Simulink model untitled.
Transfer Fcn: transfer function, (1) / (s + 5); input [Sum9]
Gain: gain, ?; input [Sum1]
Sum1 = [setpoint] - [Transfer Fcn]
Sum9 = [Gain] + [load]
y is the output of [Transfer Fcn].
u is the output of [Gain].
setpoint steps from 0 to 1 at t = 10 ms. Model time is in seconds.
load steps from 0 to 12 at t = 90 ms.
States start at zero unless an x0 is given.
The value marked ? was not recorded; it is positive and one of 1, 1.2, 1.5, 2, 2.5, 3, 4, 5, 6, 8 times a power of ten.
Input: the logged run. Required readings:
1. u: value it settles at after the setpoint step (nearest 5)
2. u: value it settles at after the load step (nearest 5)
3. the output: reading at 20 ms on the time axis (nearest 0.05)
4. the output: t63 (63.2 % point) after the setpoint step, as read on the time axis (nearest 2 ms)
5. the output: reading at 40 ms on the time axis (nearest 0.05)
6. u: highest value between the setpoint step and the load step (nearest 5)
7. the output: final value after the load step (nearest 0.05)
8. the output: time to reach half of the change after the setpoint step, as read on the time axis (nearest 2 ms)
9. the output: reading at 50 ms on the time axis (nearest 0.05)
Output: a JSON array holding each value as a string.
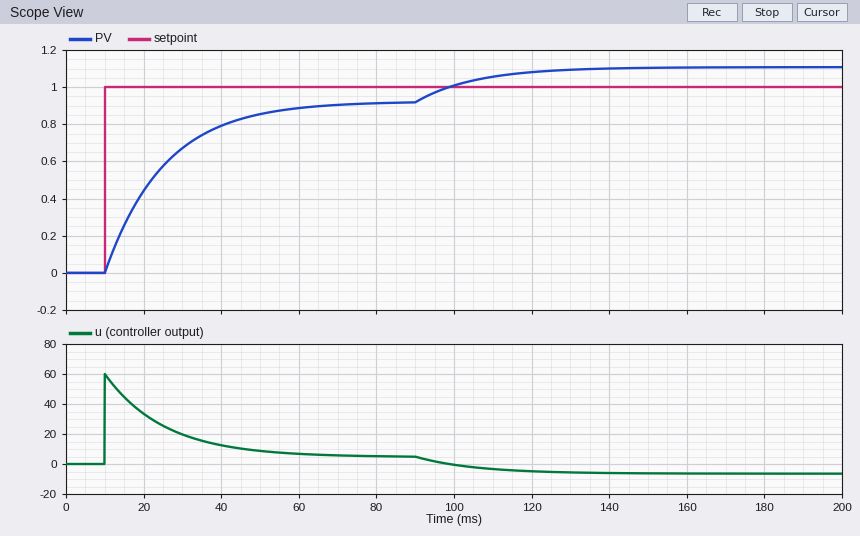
["5", "-5", "0.45", "26 ms", "0.80", "60", "1.10", "20 ms", "0.85"]
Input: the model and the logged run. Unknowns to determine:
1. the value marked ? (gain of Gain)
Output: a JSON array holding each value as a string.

["60"]
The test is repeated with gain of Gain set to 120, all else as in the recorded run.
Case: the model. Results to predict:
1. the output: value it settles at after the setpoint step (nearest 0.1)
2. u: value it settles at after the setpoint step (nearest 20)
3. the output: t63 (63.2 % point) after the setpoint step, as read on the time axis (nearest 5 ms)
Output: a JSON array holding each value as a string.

["1.0", "0", "20 ms"]
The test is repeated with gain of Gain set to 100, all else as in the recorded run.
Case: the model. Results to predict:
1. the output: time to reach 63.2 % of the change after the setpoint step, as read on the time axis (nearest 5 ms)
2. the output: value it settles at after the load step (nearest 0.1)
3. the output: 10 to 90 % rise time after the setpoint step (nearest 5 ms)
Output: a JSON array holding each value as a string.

["20 ms", "1.1", "20 ms"]
